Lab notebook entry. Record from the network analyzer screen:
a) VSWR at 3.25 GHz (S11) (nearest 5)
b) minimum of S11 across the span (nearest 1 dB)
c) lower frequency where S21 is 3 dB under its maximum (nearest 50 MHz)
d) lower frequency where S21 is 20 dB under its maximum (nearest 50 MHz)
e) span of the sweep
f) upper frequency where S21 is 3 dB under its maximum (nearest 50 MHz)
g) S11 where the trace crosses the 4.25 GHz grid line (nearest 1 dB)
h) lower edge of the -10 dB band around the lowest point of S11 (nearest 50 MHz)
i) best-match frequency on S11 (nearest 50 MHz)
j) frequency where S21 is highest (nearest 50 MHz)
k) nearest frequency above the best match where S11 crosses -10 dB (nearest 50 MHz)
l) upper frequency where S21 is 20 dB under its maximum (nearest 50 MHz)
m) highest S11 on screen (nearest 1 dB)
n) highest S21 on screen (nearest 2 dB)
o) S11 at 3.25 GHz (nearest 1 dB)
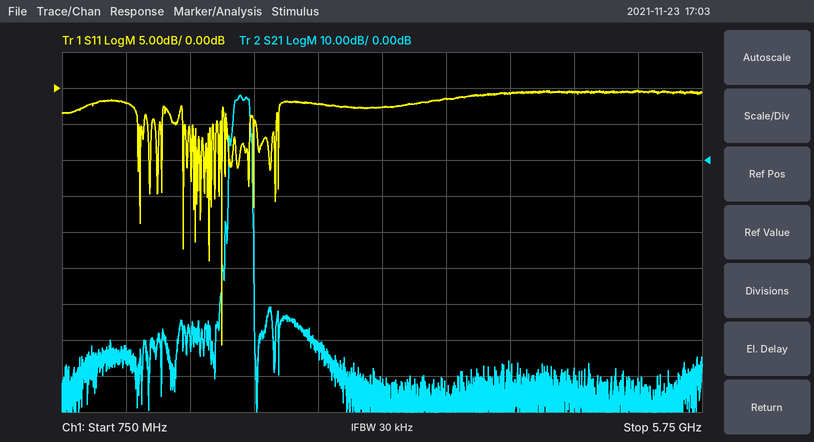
5
-36 dB
2.10 GHz
2.05 GHz
5 GHz
2.20 GHz
-1 dB
2.00 GHz
2.00 GHz
2.15 GHz
2.00 GHz
2.25 GHz
0 dB
18 dB
-3 dB
